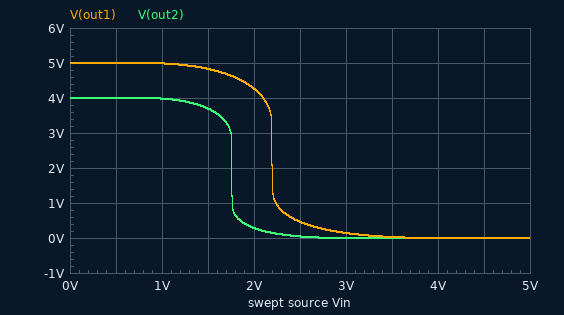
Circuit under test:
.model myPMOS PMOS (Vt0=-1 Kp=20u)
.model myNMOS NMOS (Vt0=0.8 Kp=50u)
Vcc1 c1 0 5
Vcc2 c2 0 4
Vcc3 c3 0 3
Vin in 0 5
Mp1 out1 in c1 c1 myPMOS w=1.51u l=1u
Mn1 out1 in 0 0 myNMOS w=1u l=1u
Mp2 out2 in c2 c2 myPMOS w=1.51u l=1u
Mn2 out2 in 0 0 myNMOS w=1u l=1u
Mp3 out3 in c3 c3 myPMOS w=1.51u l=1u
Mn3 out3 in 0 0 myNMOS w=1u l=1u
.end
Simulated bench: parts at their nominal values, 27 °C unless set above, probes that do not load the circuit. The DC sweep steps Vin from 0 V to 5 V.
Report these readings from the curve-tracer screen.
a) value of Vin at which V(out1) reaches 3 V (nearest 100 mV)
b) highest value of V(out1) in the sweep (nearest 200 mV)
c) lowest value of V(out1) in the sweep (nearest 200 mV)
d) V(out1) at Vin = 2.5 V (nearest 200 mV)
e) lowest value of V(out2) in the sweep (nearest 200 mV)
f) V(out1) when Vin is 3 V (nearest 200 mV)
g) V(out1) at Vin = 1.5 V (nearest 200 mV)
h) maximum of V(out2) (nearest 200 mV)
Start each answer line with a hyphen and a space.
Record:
- 2.2 V
- 5.0 V
- 0 V
- 400 mV
- 0 V
- 200 mV
- 4.8 V
- 4.0 V
